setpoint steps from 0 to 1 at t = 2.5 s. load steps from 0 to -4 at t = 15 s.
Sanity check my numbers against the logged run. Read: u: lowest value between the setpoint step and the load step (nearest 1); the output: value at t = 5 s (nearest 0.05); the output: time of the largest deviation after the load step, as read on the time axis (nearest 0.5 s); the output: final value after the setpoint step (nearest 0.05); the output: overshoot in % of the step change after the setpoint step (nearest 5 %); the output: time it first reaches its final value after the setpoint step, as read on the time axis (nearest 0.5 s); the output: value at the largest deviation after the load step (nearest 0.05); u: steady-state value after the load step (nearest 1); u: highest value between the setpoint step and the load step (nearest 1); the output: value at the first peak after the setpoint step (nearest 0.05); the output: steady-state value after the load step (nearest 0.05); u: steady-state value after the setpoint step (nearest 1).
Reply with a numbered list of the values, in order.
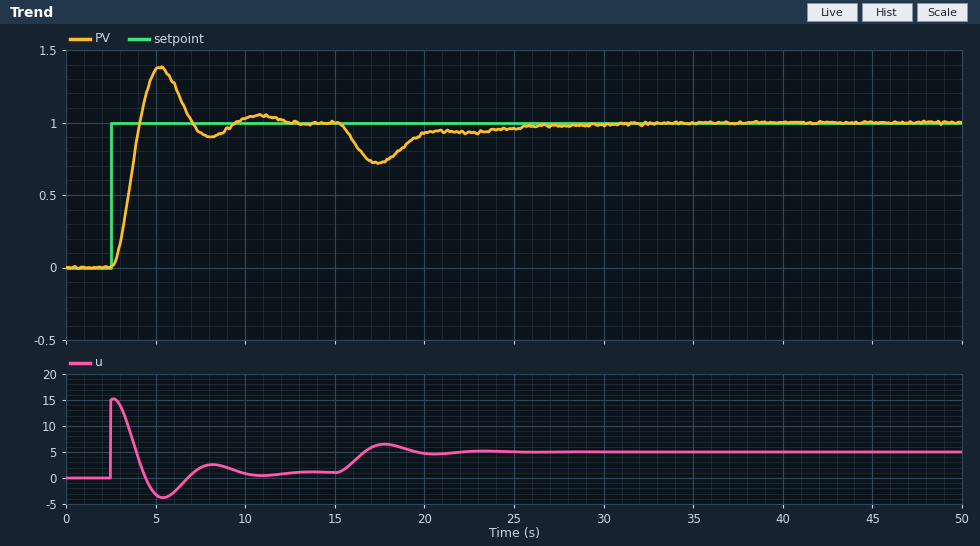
1. -4
2. 1.35
3. 17.5 s
4. 1.00
5. 40 %
6. 4.0 s
7. 0.70
8. 5
9. 15
10. 1.40
11. 1.00
12. 1
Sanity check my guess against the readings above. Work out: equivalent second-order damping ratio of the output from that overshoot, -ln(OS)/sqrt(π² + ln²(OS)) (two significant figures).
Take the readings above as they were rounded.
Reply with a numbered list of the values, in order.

1. 0.28
